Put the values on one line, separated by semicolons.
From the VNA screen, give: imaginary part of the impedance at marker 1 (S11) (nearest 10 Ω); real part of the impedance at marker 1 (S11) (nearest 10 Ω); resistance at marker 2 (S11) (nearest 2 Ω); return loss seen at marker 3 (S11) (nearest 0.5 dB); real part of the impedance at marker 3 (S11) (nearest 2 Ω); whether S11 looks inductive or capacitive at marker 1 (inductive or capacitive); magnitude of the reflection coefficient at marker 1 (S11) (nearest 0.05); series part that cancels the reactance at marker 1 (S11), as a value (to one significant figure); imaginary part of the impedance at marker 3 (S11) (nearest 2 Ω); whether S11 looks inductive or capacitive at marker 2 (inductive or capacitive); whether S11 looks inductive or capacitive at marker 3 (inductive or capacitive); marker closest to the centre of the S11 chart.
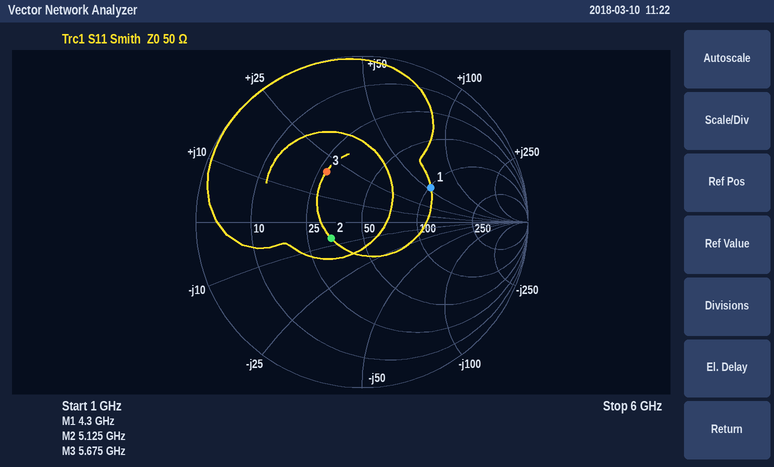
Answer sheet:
+50 Ω; 100 Ω; 34 Ω; 8.5 dB; 28 Ω; inductive; 0.45; 700 fF; +20 Ω; capacitive; inductive; marker 2
